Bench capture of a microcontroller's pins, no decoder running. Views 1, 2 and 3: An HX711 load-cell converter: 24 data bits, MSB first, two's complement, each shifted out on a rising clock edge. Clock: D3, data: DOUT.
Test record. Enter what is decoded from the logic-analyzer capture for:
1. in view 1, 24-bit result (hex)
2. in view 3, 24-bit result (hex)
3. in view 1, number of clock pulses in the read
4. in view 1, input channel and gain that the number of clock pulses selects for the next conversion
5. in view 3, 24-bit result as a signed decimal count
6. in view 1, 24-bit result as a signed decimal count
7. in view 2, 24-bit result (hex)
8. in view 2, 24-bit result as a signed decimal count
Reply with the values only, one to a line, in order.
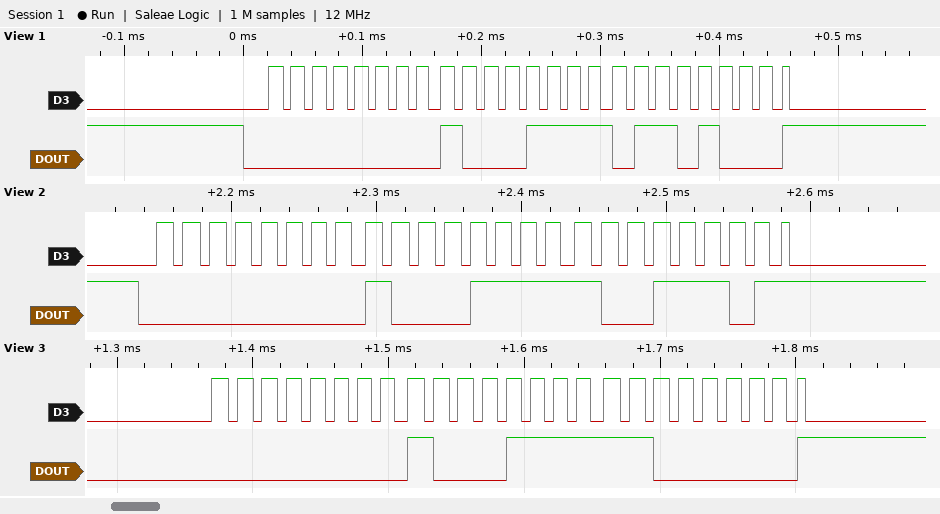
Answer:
0x008F68
0x008FC0
25
channel A, gain 128
36800
36712
0x008F9D
36765
